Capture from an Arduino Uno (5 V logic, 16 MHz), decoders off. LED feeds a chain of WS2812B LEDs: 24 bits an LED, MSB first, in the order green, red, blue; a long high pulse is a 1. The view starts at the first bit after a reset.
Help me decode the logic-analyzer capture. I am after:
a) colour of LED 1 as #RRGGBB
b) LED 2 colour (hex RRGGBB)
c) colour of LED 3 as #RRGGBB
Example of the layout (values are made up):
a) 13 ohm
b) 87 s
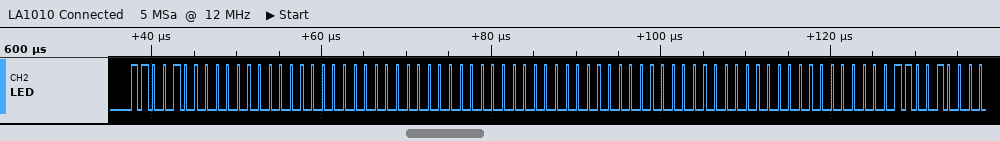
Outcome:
a) #00C800
b) #000000
c) #000000
